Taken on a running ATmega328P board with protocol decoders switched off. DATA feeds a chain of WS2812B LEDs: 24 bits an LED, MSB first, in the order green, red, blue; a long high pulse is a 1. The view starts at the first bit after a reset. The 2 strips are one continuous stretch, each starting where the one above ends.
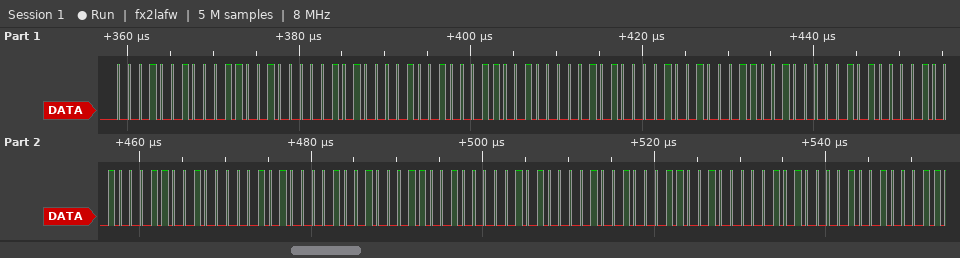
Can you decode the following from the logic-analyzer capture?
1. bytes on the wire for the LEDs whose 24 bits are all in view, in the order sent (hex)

12 32 0A 12 32 0A 12 32 0A 12 32 0A 12 32 0A 12 32 0A
